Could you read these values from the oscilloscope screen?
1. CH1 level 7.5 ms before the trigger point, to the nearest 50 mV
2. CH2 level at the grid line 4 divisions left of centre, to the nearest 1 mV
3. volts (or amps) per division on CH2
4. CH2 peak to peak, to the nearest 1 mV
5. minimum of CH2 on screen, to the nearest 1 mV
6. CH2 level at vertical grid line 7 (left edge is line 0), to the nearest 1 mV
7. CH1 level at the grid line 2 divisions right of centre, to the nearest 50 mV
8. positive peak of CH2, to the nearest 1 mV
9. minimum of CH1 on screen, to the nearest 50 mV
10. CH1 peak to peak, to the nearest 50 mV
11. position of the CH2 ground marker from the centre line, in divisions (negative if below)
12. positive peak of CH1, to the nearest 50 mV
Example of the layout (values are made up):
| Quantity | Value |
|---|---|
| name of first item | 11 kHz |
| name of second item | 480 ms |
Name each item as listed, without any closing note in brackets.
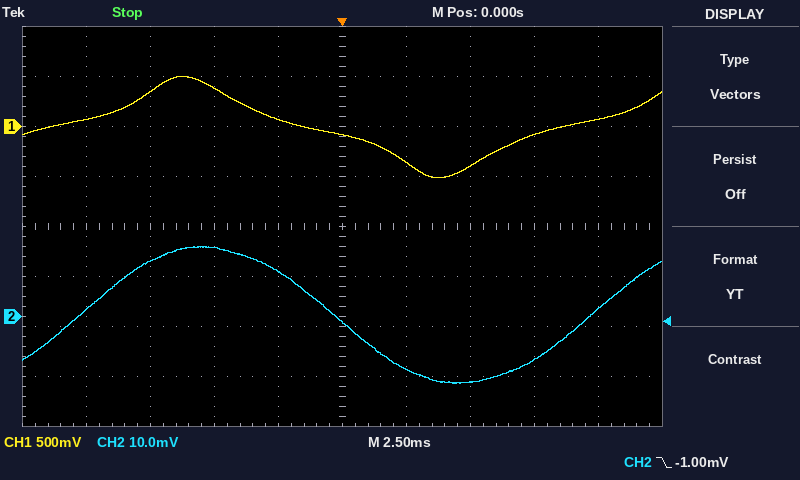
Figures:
| Quantity | Value |
|---|---|
| CH1 level 7.5 ms before the trigger point, to the nearest 50 mV | 350 mV |
| CH2 level at the grid line 4 divisions left of centre, to the nearest 1 mV | 1 mV |
| volts (or amps) per division on CH2 | 10 mV |
| CH2 peak to peak, to the nearest 1 mV | 27 mV |
| minimum of CH2 on screen, to the nearest 1 mV | -13 mV |
| CH2 level at vertical grid line 7 (left edge is line 0), to the nearest 1 mV | -13 mV |
| CH1 level at the grid line 2 divisions right of centre, to the nearest 50 mV | -400 mV |
| positive peak of CH2, to the nearest 1 mV | 14 mV |
| minimum of CH1 on screen, to the nearest 50 mV | -500 mV |
| CH1 peak to peak, to the nearest 50 mV | 1.00 V |
| position of the CH2 ground marker from the centre line, in divisions | -1.8 div |
| positive peak of CH1, to the nearest 50 mV | 500 mV |
